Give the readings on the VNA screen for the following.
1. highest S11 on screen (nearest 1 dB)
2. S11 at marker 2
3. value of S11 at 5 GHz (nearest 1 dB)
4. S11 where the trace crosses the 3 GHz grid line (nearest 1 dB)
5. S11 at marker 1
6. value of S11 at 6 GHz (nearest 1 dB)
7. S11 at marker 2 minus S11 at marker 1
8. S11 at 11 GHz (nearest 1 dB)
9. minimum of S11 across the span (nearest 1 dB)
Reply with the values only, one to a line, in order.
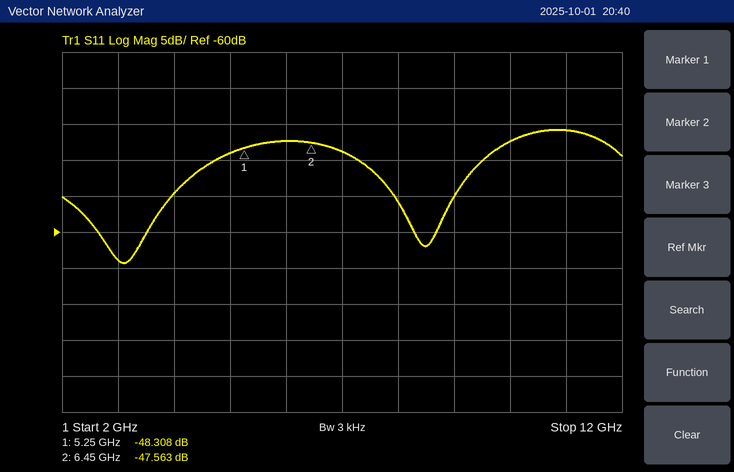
-46 dB
-47.563 dB
-49 dB
-64 dB
-48.308 dB
-47 dB
0.745 dB
-46 dB
-64 dB
